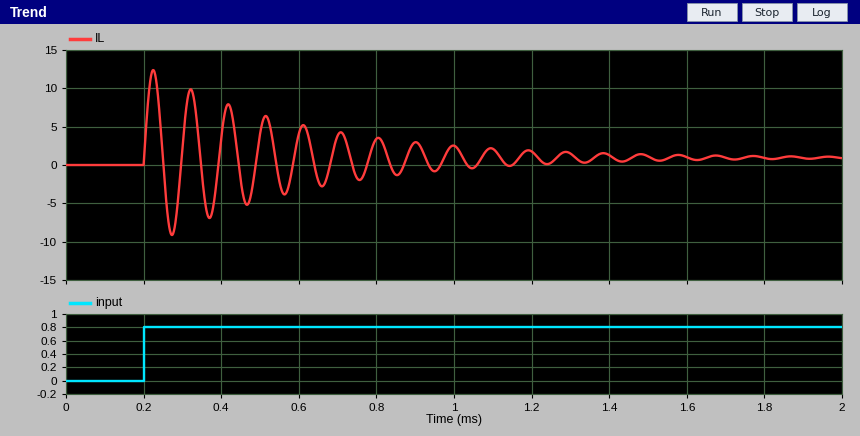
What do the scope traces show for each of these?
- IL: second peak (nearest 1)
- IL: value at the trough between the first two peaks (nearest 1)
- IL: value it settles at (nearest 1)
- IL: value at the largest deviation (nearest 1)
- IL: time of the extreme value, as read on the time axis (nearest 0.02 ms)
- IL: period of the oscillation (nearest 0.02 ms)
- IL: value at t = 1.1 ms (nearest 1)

10
-9
1
12
0.22 ms
0.10 ms
2
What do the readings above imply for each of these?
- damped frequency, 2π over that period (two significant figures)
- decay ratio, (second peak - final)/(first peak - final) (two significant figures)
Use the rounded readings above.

63 rad/ms
0.82
